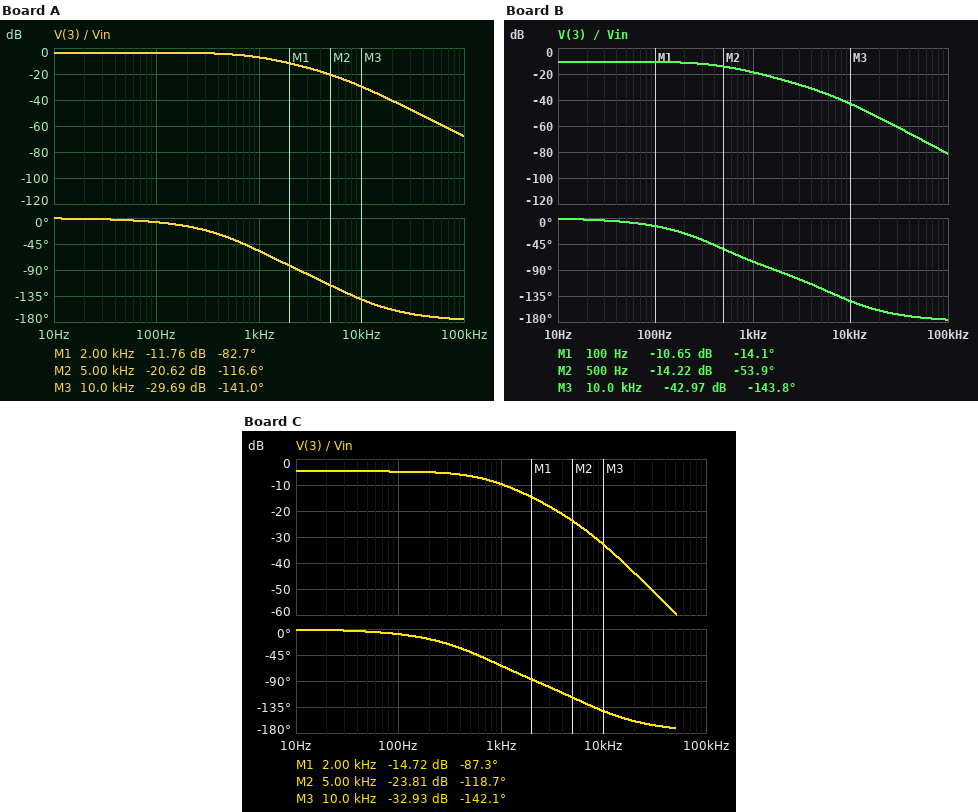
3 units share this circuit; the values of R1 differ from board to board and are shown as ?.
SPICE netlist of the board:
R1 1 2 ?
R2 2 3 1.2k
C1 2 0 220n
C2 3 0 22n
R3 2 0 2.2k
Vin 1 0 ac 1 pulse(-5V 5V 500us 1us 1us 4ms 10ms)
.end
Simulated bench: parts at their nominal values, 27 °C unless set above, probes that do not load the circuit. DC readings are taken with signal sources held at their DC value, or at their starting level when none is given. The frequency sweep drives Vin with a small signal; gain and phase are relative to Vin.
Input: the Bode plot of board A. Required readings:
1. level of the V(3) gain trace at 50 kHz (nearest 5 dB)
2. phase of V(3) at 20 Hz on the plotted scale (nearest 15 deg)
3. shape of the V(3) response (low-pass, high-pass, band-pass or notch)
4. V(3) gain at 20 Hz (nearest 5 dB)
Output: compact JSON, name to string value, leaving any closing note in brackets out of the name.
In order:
{"level of the V(3) gain trace at 50 kHz": "-55 dB", "phase of V(3) at 20 Hz on the plotted scale": "0 deg", "shape of the V(3) response": "low-pass", "V(3) gain at 20 Hz": "-5 dB"}
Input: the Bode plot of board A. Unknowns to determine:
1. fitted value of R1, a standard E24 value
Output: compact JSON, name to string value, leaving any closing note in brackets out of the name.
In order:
{"fitted value of R1, a standard E24 value": "1.1 kΩ"}
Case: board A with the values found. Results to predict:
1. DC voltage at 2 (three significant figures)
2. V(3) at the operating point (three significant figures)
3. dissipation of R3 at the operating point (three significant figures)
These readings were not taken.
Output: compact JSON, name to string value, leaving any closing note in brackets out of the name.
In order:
{"DC voltage at 2": "-3.33 V", "V(3) at the operating point": "-3.33 V", "dissipation of R3 at the operating point": "5.05 mW"}
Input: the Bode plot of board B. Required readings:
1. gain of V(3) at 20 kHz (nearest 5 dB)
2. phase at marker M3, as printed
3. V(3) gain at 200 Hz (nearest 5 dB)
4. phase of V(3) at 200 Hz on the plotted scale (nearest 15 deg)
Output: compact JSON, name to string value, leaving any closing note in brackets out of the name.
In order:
{"gain of V(3) at 20 kHz": "-55 dB", "phase at marker M3, as printed": "-143.8 deg", "V(3) gain at 200 Hz": "-10 dB", "phase of V(3) at 200 Hz on the plotted scale": "-30 deg"}
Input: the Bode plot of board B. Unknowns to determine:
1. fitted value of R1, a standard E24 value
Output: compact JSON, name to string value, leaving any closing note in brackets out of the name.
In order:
{"fitted value of R1, a standard E24 value": "5.1 kΩ"}
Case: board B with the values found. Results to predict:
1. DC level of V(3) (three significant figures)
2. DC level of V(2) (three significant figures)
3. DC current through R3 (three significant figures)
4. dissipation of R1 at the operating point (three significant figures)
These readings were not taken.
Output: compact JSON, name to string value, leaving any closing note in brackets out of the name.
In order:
{"DC level of V(3)": "-1.51 V", "DC level of V(2)": "-1.51 V", "DC current through R3": "685 µA", "dissipation of R1 at the operating point": "2.39 mW"}
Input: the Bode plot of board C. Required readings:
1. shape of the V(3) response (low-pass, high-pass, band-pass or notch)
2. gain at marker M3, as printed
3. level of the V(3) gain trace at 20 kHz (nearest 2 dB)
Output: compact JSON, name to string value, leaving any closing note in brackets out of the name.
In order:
{"shape of the V(3) response": "low-pass", "gain at marker M3, as printed": "-32.93 dB", "level of the V(3) gain trace at 20 kHz": "-44 dB"}
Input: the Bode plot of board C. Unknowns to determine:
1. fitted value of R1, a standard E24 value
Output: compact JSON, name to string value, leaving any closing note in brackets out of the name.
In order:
{"fitted value of R1, a standard E24 value": "1.6 kΩ"}
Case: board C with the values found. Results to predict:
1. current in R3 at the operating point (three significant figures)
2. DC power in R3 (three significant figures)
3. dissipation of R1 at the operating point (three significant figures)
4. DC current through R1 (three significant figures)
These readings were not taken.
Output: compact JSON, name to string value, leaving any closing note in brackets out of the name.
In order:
{"current in R3 at the operating point": "1.32 mA", "DC power in R3": "3.81 mW", "dissipation of R1 at the operating point": "2.77 mW", "DC current through R1": "1.32 mA"}
